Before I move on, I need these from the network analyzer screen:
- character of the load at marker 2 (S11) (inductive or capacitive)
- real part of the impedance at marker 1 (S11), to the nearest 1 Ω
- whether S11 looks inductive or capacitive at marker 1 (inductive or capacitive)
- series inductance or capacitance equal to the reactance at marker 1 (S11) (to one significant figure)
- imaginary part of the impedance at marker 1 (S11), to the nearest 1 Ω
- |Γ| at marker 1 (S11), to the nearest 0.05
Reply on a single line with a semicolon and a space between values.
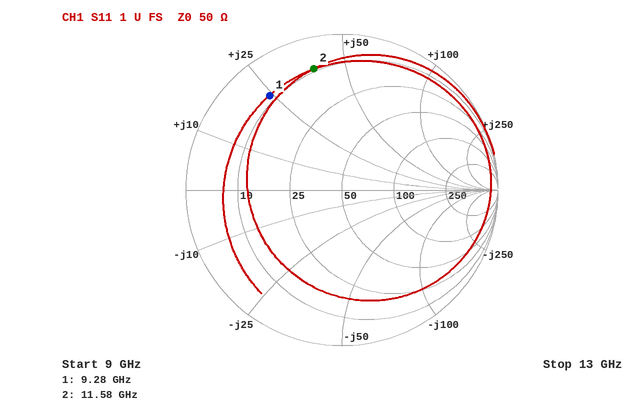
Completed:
inductive; 8 Ω; inductive; 400 pH; +24 Ω; 0.75
